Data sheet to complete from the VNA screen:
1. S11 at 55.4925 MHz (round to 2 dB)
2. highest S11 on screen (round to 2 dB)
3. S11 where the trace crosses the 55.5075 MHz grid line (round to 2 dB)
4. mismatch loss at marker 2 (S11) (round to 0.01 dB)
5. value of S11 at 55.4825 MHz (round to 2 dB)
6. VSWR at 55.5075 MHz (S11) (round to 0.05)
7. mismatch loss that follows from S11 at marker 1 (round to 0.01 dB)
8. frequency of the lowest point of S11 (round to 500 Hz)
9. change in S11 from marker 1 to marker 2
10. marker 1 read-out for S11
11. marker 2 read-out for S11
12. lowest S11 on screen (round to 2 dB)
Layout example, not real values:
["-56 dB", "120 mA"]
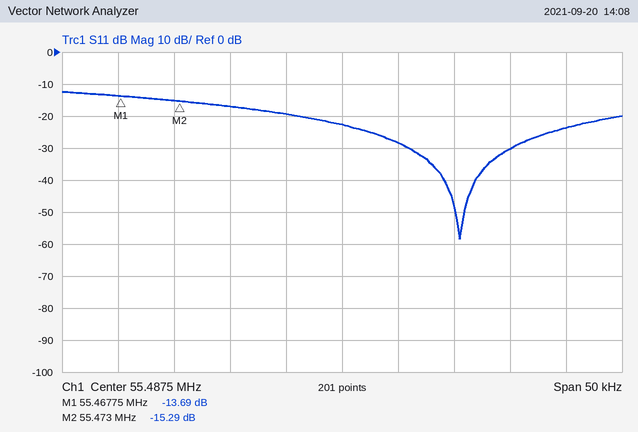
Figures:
["-28 dB", "-12 dB", "-24 dB", "0.13 dB", "-20 dB", "1.15", "0.19 dB", "55.4980 MHz", "-1.60 dB", "-13.69 dB", "-15.29 dB", "-58 dB"]
